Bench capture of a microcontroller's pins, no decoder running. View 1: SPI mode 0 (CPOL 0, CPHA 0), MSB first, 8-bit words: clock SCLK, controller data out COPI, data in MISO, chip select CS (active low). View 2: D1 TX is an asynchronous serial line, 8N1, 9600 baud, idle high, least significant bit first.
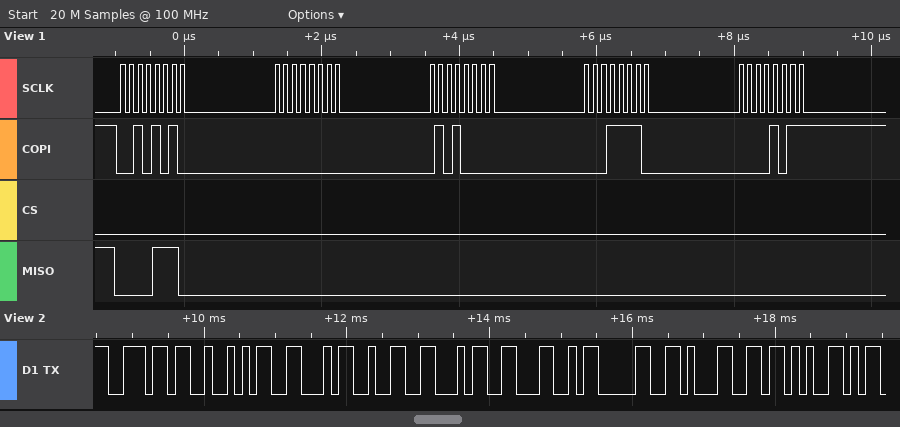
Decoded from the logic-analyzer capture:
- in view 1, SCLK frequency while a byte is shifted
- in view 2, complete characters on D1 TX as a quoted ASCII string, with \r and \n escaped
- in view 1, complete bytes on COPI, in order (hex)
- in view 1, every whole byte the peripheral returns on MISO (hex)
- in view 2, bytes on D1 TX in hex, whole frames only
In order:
8 MHz
"nRF24L01+"
2A 00 50 1E 0B
0E 00 00 00 00
0x6E 0x52 0x46 0x32 0x34 0x4C 0x30 0x31 0x2B
